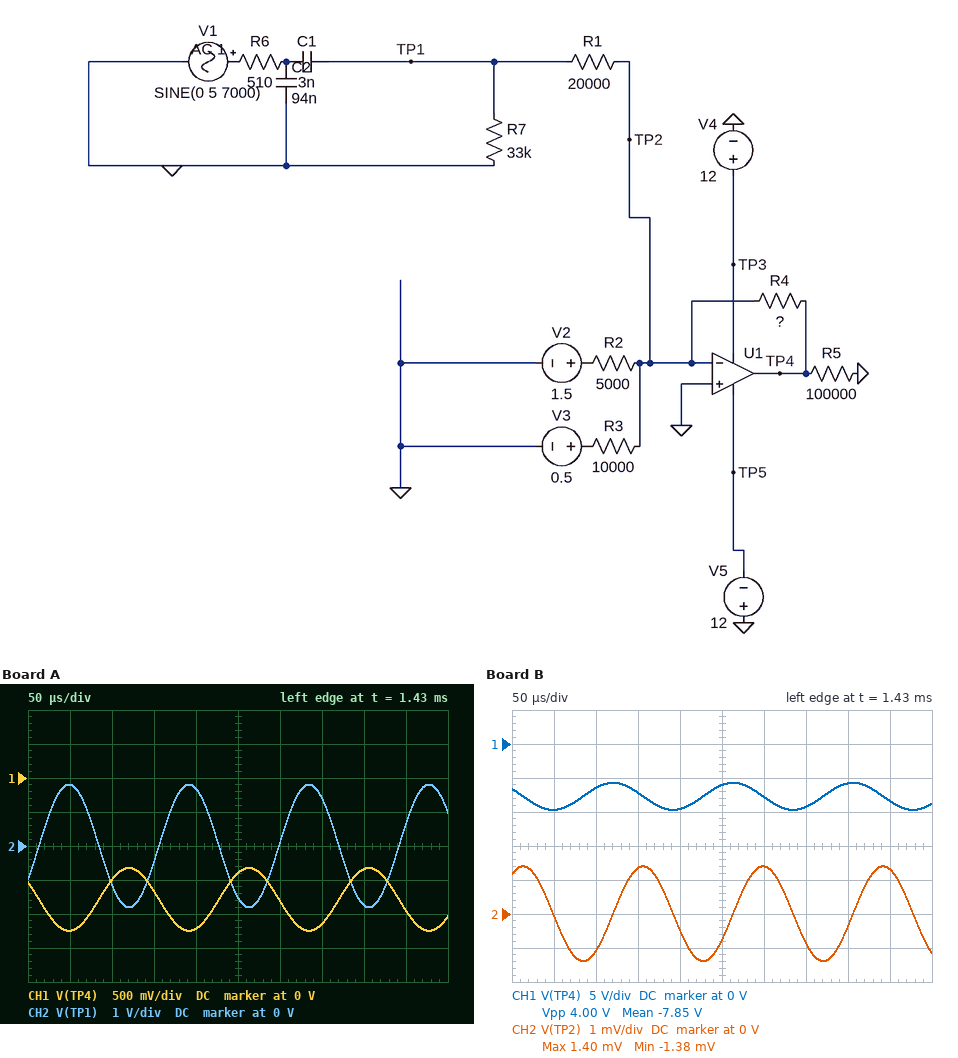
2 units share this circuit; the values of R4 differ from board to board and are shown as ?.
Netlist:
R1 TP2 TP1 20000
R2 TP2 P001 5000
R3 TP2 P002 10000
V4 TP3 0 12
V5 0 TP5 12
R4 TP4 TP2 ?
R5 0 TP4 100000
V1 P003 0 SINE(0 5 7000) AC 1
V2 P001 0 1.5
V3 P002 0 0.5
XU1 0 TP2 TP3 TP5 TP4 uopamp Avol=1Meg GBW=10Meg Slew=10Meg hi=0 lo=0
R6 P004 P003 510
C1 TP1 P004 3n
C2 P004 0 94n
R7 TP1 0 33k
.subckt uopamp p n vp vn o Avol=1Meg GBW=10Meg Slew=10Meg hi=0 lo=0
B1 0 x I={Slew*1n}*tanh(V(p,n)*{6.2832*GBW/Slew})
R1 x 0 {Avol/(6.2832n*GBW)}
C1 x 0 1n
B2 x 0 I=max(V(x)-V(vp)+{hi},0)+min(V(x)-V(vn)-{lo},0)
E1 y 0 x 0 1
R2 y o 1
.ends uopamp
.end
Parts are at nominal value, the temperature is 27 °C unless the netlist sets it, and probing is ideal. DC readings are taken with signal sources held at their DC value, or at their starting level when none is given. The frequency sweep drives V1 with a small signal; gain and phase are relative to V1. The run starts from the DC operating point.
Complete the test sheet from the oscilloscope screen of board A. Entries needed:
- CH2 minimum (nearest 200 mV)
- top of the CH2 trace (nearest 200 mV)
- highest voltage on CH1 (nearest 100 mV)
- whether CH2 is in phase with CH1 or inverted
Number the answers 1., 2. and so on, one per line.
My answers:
1. -1.8 V
2. 1.8 V
3. -1.3 V
4. inverted
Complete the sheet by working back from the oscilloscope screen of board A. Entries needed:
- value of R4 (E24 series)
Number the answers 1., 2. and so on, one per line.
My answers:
1. 5.1 kΩ
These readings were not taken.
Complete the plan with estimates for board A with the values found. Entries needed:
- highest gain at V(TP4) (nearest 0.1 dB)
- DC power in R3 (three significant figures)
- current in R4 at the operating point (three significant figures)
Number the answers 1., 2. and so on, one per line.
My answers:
1. -19.2 dB
2. 25.0 µW
3. 350 µA
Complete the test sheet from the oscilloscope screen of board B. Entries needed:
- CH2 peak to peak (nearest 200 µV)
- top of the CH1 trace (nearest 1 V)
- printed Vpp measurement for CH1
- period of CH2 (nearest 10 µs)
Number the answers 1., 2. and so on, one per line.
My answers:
1. 2.8 mV
2. -6 V
3. 4.00 V
4. 140 µs
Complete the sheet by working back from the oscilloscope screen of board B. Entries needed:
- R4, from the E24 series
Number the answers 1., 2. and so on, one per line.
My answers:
1. 22 kΩ
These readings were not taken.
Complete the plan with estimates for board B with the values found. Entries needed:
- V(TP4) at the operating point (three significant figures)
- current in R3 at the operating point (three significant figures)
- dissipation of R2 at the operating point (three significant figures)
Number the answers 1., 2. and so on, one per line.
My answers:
1. -7.70 V
2. 50.0 µA
3. 450 µW
